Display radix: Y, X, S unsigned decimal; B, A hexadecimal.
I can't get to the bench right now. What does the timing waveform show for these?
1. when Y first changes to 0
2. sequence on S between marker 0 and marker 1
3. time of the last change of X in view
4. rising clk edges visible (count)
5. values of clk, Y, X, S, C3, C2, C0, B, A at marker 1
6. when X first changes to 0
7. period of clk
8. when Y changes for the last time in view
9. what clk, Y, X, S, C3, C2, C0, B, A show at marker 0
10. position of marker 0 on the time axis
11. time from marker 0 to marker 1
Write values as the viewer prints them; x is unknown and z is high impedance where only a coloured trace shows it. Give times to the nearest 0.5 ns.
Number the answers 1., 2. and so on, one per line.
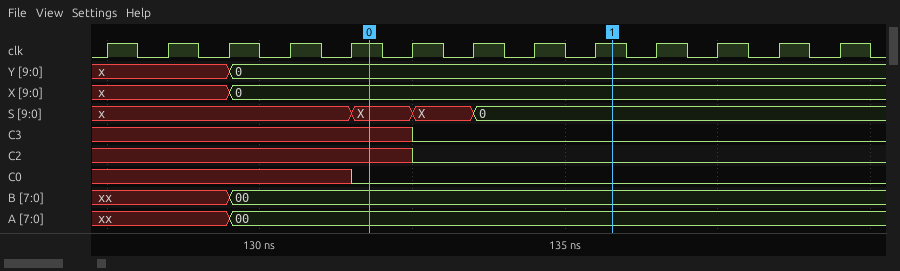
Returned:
1. 129.5 ns
2. X, X, 0
3. 129.5 ns
4. 13
5. clk=1, Y=0, X=0, S=0, C3=0, C2=0, C0=0, B=00, A=00
6. 129.5 ns
7. 1 ns
8. 129.5 ns
9. clk=1, Y=0, X=0, S=X, C3=x, C2=x, C0=0, B=00, A=00
10. 132 ns
11. 4 ns
